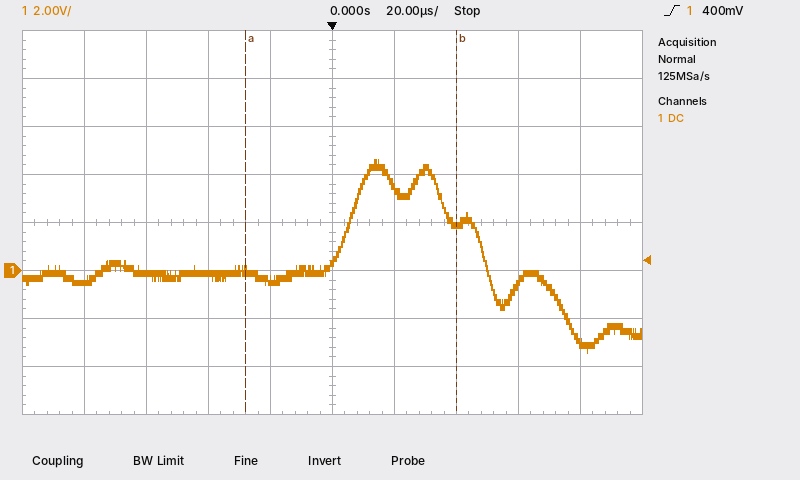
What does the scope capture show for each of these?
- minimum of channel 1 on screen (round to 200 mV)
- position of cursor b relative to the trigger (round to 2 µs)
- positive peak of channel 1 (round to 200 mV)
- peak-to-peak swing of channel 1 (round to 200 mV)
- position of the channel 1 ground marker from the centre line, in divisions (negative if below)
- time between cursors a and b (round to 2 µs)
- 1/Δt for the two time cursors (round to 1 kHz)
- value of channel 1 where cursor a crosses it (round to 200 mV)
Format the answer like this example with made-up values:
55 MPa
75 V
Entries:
-3.4 V
+40 µs
4.6 V
8.0 V
-1.0 div
68 µs
15 kHz
0.0 V
